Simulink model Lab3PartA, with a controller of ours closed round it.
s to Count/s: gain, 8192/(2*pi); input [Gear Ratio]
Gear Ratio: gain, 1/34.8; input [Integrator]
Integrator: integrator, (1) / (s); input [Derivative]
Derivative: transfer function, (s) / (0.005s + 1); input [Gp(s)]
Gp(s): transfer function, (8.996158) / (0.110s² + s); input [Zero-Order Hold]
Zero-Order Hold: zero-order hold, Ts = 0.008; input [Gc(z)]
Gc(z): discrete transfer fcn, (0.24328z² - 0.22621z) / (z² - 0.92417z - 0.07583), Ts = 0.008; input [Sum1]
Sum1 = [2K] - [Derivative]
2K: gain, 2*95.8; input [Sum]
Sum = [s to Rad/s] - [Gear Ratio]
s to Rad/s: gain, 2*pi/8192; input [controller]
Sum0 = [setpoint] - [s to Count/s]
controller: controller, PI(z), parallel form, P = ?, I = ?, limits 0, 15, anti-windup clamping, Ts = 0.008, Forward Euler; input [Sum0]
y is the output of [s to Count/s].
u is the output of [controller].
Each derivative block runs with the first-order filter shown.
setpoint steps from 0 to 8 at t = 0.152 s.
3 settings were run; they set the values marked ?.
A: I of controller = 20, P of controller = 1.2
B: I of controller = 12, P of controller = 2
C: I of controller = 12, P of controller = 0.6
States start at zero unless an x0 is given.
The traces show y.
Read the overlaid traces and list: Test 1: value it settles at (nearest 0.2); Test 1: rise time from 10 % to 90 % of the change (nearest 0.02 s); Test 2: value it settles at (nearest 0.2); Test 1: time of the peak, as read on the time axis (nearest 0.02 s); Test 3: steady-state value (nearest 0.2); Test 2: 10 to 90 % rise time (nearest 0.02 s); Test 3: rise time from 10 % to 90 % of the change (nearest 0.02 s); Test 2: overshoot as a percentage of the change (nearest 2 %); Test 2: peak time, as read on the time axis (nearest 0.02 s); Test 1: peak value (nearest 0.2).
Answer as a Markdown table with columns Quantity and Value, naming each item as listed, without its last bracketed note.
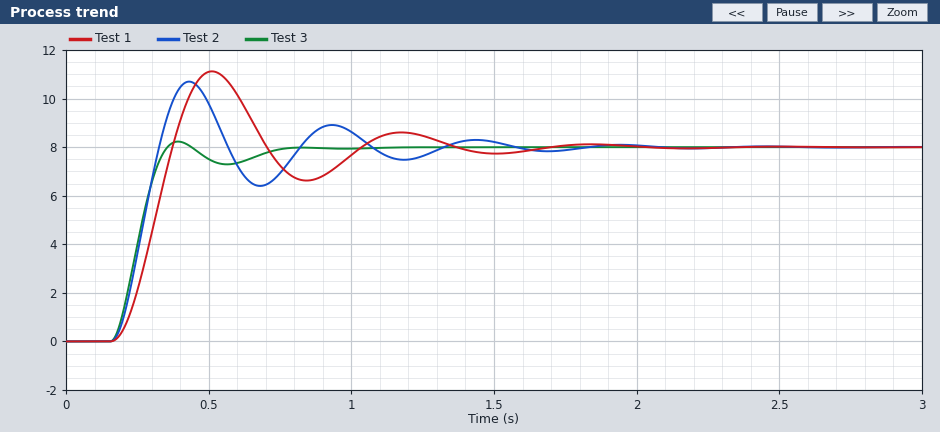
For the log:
| Quantity | Value |
|---|---|
| Test 1: value it settles at | 8.0 |
| Test 1: rise time from 10 % to 90 % of the change | 0.14 s |
| Test 2: value it settles at | 8.0 |
| Test 1: time of the peak, as read on the time axis | 0.52 s |
| Test 3: steady-state value | 8.0 |
| Test 2: 10 to 90 % rise time | 0.12 s |
| Test 3: rise time from 10 % to 90 % of the change | 0.12 s |
| Test 2: overshoot as a percentage of the change | 34 % |
| Test 2: peak time, as read on the time axis | 0.44 s |
| Test 1: peak value | 11.2 |
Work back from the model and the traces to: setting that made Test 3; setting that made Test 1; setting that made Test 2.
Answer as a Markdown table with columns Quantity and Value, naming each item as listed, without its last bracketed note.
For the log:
| Quantity | Value |
|---|---|
| setting that made Test 3 | B |
| setting that made Test 1 | C |
| setting that made Test 2 | A |
